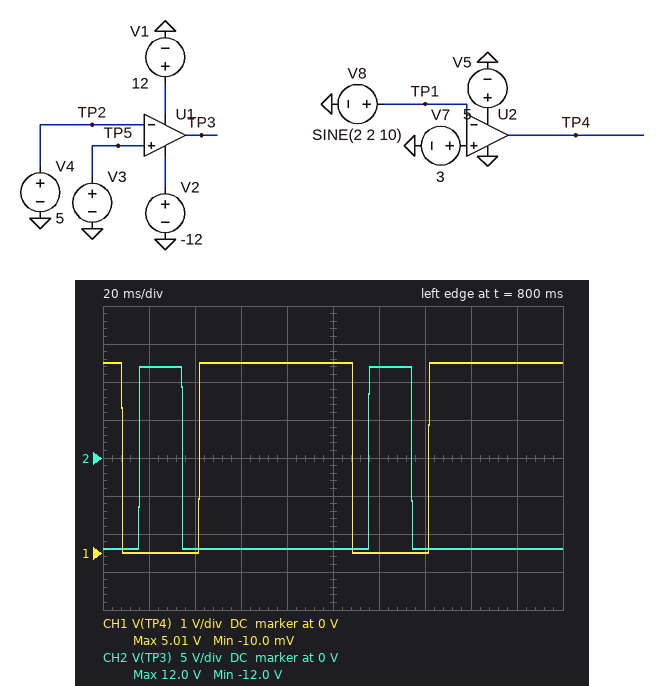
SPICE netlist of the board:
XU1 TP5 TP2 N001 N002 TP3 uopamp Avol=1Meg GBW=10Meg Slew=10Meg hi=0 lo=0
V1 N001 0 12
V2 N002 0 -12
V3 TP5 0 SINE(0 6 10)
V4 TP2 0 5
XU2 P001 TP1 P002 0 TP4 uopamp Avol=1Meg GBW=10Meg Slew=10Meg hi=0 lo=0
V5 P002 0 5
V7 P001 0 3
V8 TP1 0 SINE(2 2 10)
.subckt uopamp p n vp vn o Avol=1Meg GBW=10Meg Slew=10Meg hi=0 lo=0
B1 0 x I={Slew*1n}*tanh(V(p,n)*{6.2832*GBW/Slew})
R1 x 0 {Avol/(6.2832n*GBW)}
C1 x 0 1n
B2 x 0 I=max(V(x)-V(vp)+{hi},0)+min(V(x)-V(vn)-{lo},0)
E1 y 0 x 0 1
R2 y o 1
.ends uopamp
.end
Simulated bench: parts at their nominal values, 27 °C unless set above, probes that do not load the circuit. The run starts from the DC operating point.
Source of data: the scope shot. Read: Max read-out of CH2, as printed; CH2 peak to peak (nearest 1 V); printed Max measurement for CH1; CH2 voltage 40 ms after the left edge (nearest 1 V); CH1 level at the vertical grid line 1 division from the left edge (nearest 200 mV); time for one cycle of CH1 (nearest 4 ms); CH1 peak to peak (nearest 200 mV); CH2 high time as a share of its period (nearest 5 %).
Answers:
12.0 V
24 V
5.01 V
-12 V
0 V
100 ms
5.0 V
20 %
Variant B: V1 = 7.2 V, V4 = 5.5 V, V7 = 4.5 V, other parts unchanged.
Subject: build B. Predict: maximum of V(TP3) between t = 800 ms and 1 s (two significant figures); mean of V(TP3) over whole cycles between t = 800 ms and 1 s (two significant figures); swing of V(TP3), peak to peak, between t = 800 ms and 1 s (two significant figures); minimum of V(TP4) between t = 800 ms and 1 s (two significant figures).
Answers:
7.2 V
-9.5 V
19 V
5.0 V
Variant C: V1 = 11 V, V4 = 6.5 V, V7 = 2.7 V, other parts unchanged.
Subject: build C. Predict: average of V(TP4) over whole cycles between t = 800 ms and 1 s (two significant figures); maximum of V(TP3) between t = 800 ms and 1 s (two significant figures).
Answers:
3.1 V
-12 V
